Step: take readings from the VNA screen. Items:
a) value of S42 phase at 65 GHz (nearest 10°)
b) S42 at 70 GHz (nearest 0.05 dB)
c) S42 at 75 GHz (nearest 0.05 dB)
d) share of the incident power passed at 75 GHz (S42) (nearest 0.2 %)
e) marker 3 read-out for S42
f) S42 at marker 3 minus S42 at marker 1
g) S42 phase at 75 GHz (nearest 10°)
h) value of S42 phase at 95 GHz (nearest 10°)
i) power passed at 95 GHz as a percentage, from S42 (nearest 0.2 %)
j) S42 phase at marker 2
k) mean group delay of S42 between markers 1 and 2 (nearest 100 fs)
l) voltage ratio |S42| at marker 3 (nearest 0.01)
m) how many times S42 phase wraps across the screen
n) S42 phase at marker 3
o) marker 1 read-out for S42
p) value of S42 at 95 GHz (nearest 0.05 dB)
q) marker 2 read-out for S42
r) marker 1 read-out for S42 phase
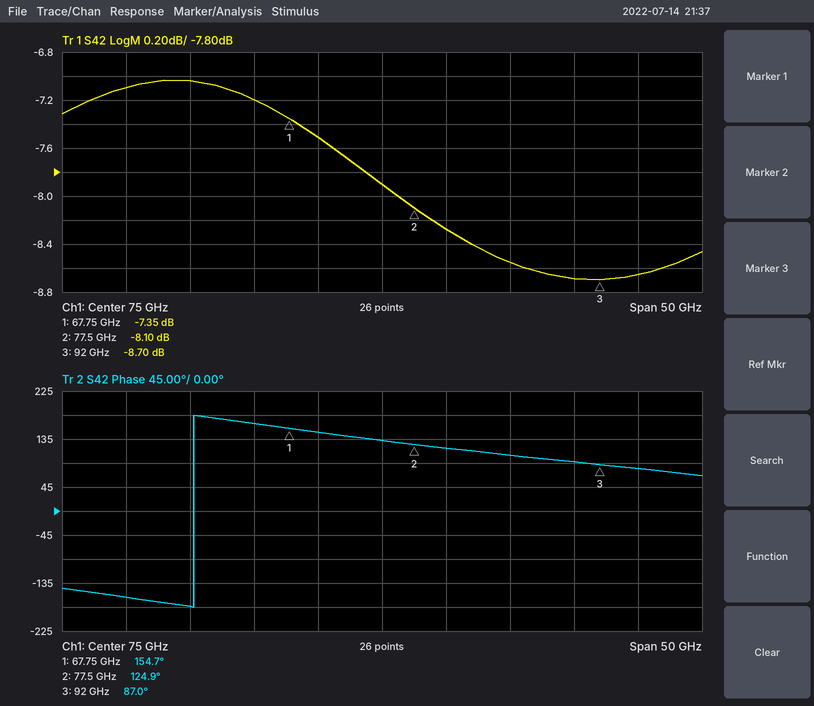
160°
-7.50 dB
-7.90 dB
16.2 %
-8.70 dB
-1.35 dB
130°
80°
13.6 %
124.9°
8.5 ps
0.37
1
87.0°
-7.35 dB
-8.65 dB
-8.10 dB
154.7°
